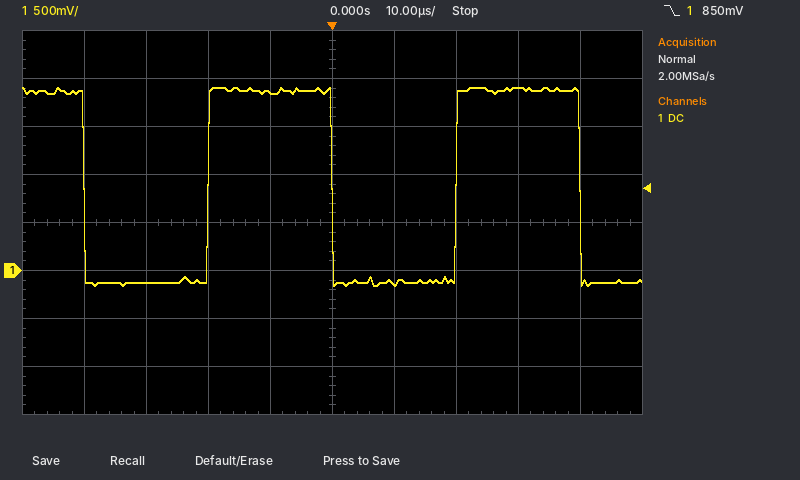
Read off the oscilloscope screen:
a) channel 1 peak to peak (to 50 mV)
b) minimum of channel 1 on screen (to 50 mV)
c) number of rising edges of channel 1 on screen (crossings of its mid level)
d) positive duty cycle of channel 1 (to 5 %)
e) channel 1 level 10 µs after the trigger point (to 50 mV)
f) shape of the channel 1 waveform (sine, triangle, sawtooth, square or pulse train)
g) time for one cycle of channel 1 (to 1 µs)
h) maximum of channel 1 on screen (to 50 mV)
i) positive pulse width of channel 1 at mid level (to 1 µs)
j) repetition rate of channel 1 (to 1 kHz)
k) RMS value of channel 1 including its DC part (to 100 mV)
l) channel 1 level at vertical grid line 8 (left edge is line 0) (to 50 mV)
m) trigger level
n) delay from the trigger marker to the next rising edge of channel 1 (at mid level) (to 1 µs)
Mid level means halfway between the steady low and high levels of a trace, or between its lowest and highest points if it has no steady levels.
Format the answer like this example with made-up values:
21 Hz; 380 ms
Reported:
2.05 V; -150 mV; 2; 50 %; -150 mV; square; 40 µs; 1.90 V; 20 µs; 25 kHz; 1.3 V; 1.90 V; 850 mV; 20 µs
